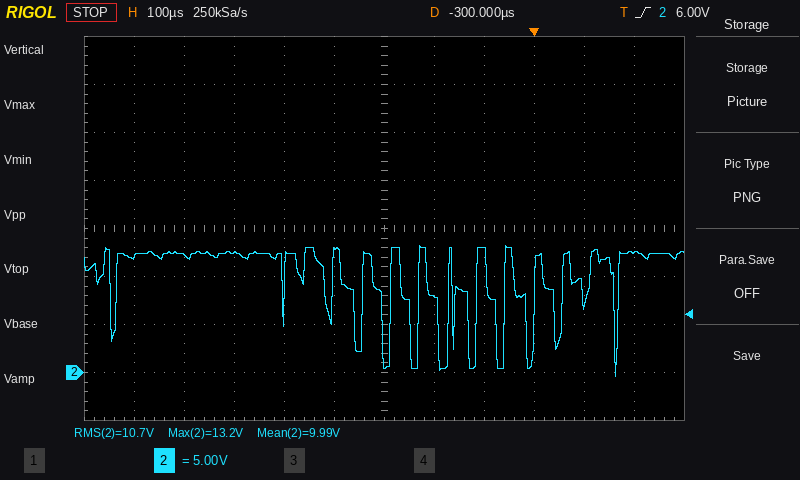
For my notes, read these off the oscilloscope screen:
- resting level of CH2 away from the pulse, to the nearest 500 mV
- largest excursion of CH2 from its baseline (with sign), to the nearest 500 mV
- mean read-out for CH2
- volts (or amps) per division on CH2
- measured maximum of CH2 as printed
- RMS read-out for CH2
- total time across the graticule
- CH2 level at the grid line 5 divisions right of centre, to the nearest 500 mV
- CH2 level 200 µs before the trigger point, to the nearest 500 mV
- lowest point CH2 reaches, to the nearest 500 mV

12.5 V
-13.0 V
9.99 V
5 V
13.2 V
10.7 V
1.2 ms
12.5 V
8.0 V
-500 mV
